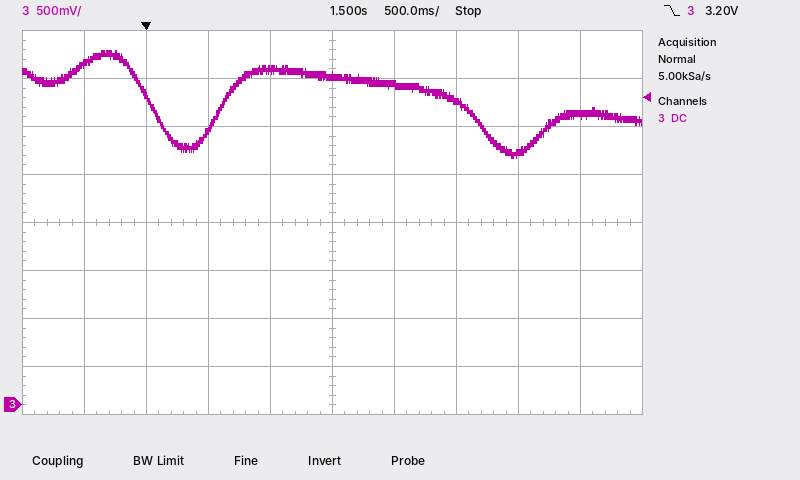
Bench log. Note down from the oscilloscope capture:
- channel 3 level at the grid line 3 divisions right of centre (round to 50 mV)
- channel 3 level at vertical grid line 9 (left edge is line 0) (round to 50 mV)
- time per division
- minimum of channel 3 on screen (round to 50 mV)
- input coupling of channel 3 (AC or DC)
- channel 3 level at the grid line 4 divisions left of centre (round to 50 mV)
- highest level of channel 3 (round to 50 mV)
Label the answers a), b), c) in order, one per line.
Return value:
a) 2.60 V
b) 3.00 V
c) 500 ms
d) 2.55 V
e) DC
f) 3.55 V
g) 3.70 V
